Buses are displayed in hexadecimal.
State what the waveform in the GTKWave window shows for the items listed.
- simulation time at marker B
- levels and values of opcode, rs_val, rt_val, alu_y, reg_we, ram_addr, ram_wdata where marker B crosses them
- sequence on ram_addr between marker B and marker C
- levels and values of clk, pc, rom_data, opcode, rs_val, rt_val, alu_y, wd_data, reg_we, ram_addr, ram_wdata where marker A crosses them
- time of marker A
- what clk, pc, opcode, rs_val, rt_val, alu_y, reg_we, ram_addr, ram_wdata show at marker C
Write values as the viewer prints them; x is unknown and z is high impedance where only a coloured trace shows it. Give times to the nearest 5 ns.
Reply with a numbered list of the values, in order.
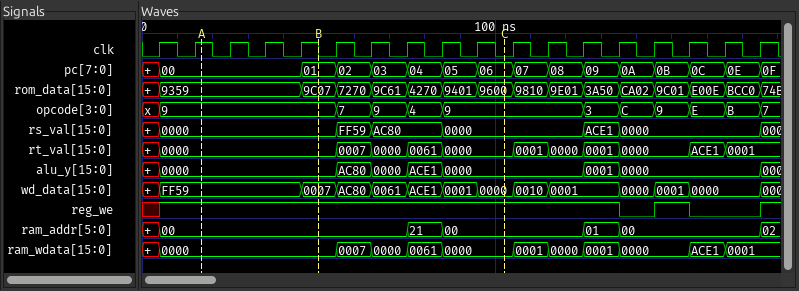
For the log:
1. 50 ns
2. opcode=9, rs_val=0000, rt_val=0000, alu_y=0000, reg_we=1, ram_addr=00, ram_wdata=0000
3. 00, 21, 00
4. clk=1, pc=00, rom_data=9359, opcode=9, rs_val=0000, rt_val=0000, alu_y=0000, wd_data=FF59, reg_we=1, ram_addr=00, ram_wdata=0000
5. 15 ns
6. clk=0, pc=06, opcode=9, rs_val=0000, rt_val=0000, alu_y=0000, reg_we=1, ram_addr=00, ram_wdata=0000
